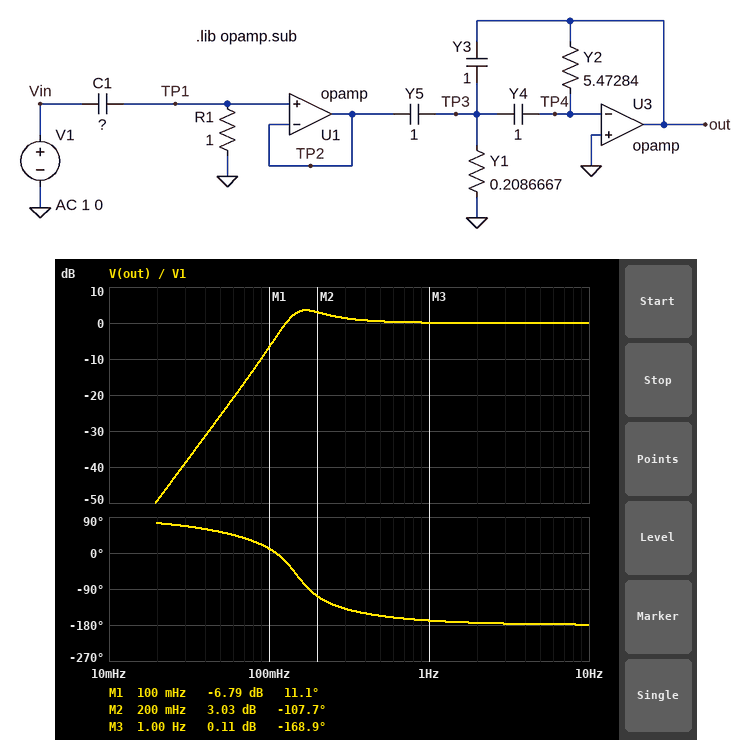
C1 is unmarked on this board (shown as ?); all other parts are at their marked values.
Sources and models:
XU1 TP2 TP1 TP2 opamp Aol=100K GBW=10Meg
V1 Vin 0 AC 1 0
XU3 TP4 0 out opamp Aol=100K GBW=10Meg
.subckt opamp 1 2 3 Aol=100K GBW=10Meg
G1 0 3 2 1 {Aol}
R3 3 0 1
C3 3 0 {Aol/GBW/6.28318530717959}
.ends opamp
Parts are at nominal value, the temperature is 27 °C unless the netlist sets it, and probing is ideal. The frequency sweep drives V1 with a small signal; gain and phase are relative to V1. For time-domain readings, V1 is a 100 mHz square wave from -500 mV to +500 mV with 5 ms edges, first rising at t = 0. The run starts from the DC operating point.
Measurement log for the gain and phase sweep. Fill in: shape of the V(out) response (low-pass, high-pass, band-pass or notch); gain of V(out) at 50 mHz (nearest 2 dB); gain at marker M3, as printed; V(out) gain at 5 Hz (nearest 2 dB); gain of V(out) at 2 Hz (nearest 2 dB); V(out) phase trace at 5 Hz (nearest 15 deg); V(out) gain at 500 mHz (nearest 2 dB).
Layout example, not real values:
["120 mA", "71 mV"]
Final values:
["high-pass", "-26 dB", "0.11 dB", "0 dB", "0 dB", "-180 deg", "0 dB"]
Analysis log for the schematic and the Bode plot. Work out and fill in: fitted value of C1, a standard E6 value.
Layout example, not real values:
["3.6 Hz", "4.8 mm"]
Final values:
["1.5 F"]
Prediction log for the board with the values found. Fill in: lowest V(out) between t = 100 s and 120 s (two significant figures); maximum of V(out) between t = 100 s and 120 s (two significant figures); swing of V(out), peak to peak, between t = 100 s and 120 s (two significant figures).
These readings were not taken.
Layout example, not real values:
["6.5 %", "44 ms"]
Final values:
["-760 mV", "760 mV", "1.5 V"]
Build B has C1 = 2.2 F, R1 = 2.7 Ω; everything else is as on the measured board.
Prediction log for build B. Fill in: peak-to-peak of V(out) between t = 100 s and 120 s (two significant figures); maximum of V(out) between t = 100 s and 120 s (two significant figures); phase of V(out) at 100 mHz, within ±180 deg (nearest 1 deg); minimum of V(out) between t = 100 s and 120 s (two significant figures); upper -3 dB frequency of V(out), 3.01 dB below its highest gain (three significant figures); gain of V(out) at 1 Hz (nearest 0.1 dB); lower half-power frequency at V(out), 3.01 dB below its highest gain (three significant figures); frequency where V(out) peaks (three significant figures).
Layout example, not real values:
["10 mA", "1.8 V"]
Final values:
["1.7 V", "850 mV", "-21 deg", "-850 mV", "293 mHz", "0.2 dB", "127 mHz", "164 mHz"]
